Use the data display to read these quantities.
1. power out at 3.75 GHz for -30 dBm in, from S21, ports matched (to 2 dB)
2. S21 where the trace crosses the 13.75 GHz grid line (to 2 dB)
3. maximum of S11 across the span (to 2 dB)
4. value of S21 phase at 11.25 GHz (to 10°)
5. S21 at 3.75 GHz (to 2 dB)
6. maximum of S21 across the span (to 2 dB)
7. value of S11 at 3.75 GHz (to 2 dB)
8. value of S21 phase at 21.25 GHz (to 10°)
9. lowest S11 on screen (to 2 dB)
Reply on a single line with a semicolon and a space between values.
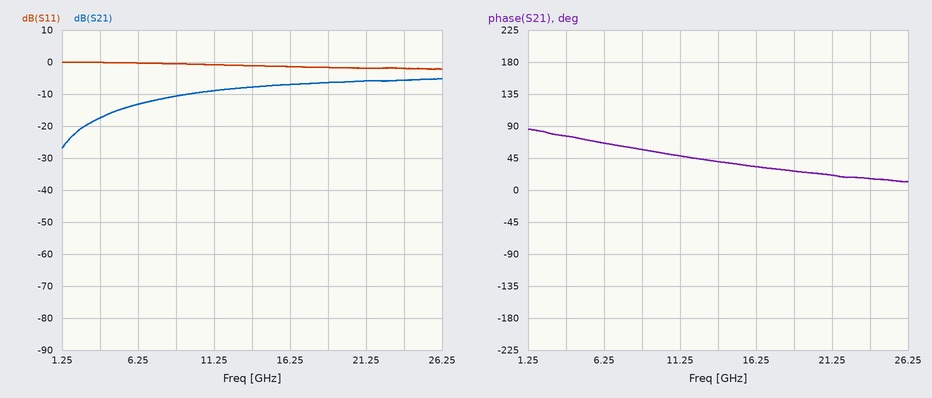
-48 dBm; -8 dB; 0 dB; 50°; -18 dB; -6 dB; 0 dB; 20°; -2 dB
